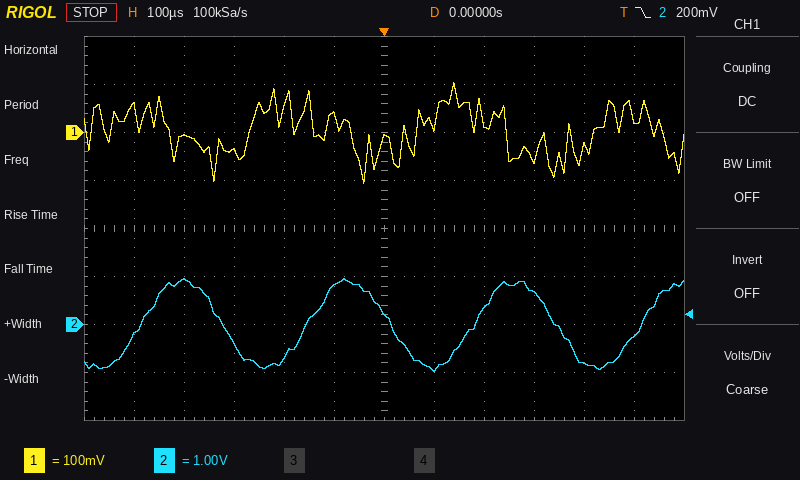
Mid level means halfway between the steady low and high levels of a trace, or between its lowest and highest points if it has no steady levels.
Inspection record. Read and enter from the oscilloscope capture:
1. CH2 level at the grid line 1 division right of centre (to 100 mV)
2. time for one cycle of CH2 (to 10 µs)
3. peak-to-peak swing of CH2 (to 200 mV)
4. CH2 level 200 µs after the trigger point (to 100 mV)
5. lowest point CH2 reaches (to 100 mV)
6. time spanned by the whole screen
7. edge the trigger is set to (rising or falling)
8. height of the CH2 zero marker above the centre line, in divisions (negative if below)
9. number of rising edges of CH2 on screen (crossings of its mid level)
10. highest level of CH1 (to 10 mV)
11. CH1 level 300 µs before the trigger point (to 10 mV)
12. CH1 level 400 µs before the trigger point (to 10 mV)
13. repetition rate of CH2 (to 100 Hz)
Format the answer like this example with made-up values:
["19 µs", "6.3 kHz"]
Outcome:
["-900 mV", "330 µs", "2.0 V", "300 mV", "-1.0 V", "1.2 ms", "falling", "-2.0 div", "4", "100 mV", "-40 mV", "-10 mV", "3.0 kHz"]
